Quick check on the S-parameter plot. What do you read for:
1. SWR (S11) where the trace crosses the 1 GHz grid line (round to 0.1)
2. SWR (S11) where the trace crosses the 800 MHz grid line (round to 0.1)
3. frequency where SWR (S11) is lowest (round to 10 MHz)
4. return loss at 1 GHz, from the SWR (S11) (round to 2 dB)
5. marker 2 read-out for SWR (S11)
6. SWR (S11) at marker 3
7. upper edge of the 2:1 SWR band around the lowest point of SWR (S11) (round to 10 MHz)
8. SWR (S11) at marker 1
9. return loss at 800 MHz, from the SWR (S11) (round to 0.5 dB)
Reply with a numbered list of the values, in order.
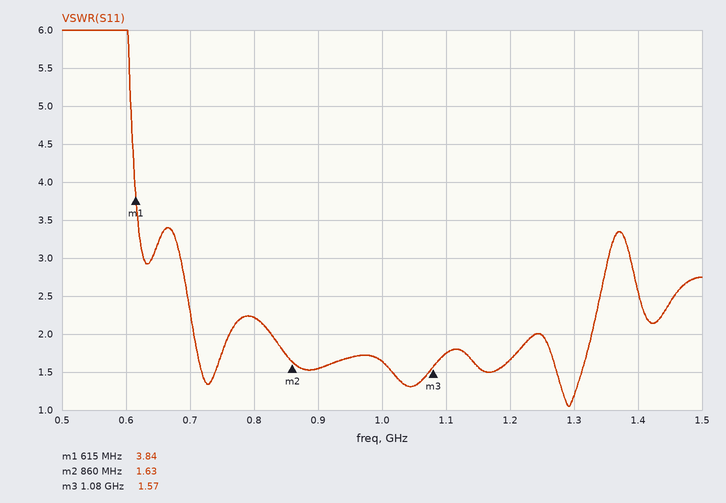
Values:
1. 1.6
2. 2.2
3. 1.29 GHz
4. 12 dB
5. 1.63
6. 1.57
7. 1.33 GHz
8. 3.84
9. 8.5 dB
